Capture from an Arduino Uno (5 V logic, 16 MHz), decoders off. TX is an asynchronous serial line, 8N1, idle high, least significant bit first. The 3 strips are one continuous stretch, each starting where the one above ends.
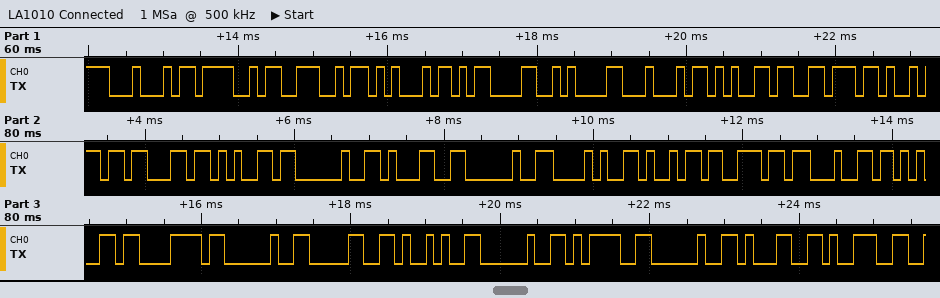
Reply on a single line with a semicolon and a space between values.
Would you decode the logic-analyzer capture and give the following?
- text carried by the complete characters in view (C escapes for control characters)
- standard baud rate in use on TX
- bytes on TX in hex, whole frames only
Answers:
"DONE\r\nDevice 1 (index 0) = 19"; 9600 baud; 44 4F 4E 45 0D 0A 44 65 76 69 63 65 20 31 20 28 69 6E 64 65 78 20 30 29 20 3D 20 31 39
